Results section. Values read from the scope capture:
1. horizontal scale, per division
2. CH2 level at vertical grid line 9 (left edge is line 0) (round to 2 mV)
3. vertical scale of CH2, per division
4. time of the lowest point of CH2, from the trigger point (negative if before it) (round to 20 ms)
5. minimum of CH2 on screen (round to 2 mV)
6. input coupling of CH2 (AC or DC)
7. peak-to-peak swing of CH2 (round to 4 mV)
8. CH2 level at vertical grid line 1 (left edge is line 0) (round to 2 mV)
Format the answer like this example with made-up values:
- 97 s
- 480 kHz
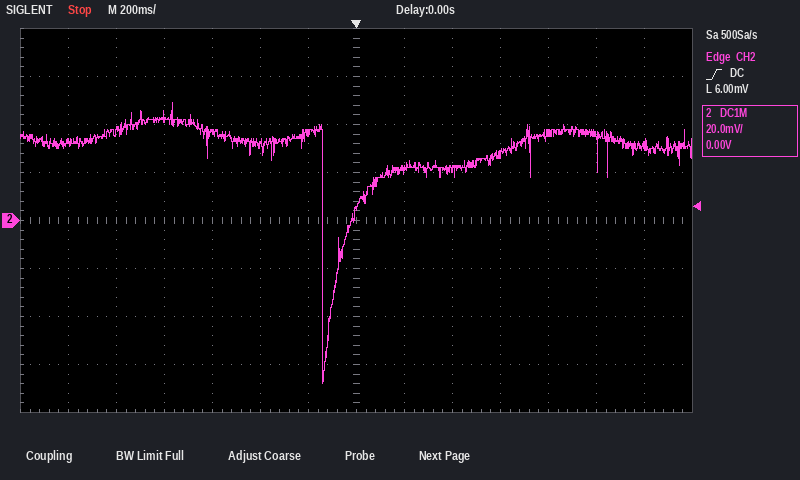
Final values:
- 200 ms
- 22 mV
- 20 mV
- -140 ms
- -68 mV
- DC
- 116 mV
- 32 mV
